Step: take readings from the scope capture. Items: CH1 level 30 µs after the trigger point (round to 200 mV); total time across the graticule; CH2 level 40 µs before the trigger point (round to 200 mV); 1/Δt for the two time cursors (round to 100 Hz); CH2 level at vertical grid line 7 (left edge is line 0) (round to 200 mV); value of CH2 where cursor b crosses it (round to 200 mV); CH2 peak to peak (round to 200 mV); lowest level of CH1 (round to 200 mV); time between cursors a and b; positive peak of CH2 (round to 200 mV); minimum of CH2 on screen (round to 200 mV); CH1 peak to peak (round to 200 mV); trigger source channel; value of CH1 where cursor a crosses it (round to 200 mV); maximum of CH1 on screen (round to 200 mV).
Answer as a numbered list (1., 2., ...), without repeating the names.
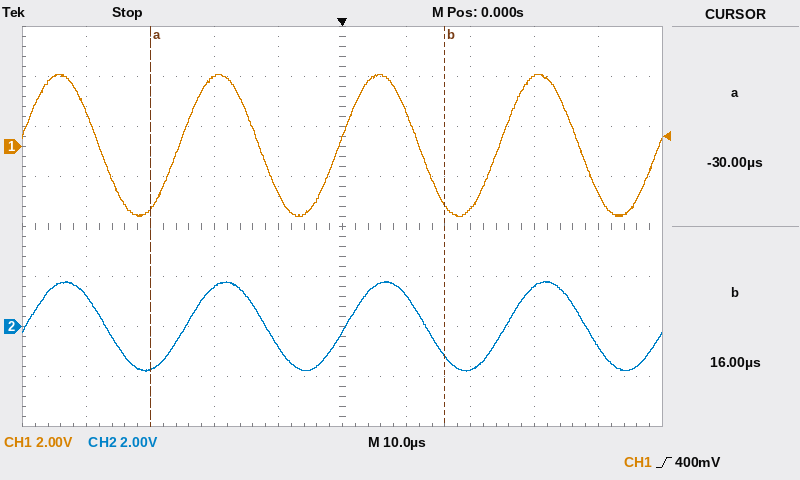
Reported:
1. 2.8 V
2. 100 µs
3. 1.2 V
4. 21.7 kHz
5. -1.8 V
6. -1.2 V
7. 3.6 V
8. -2.8 V
9. 46 µs
10. 1.8 V
11. -1.8 V
12. 5.6 V
13. CH1
14. -2.4 V
15. 2.8 V
